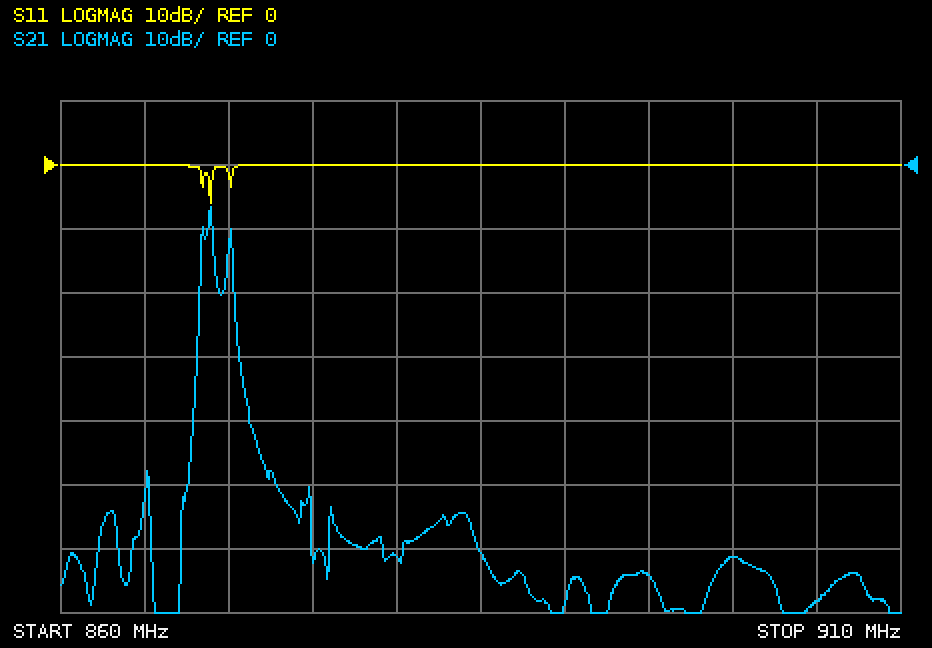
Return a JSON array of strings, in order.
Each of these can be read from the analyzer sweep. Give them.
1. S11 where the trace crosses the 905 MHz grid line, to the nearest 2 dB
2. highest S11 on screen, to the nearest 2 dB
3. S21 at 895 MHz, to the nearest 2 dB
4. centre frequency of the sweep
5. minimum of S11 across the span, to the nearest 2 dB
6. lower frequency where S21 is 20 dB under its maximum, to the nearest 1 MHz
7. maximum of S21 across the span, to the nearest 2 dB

["0 dB", "0 dB", "-64 dB", "885 MHz", "-6 dB", "868 MHz", "-6 dB"]
